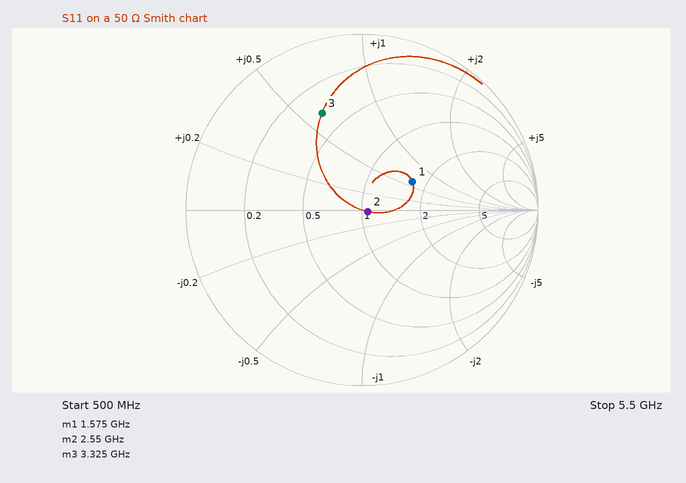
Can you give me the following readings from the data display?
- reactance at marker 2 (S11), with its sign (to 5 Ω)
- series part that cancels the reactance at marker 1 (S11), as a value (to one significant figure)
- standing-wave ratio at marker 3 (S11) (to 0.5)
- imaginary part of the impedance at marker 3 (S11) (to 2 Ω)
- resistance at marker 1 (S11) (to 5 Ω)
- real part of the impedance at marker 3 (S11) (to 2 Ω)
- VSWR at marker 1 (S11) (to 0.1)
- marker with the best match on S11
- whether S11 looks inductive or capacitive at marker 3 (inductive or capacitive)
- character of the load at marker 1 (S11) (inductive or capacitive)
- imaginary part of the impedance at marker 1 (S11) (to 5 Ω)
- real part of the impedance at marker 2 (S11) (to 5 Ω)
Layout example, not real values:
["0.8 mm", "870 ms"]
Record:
["0 Ω", "3 pF", "4.0", "+30 Ω", "85 Ω", "18 Ω", "2.0", "marker 2", "inductive", "inductive", "+30 Ω", "55 Ω"]
